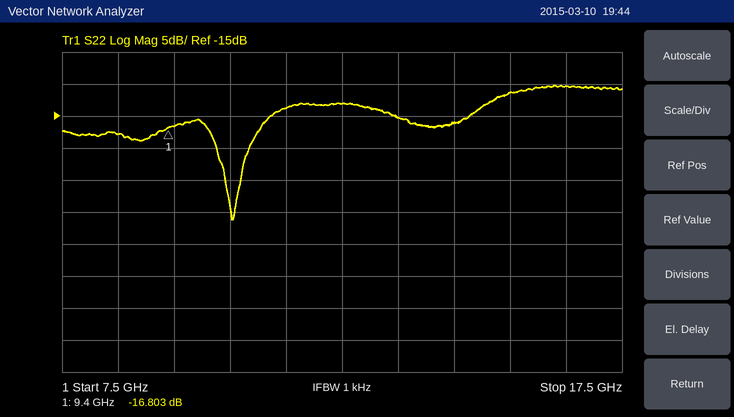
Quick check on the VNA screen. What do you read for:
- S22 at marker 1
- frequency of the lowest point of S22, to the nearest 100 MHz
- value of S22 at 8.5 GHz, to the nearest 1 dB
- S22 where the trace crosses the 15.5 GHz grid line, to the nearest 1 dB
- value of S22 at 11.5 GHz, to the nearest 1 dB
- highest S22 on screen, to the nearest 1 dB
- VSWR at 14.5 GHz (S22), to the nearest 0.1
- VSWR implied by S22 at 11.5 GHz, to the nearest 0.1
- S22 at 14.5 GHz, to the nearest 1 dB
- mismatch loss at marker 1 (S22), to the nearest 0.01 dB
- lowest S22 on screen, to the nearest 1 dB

-16.803 dB
10.5 GHz
-18 dB
-11 dB
-14 dB
-10 dB
1.4
1.5
-16 dB
0.09 dB
-31 dB
